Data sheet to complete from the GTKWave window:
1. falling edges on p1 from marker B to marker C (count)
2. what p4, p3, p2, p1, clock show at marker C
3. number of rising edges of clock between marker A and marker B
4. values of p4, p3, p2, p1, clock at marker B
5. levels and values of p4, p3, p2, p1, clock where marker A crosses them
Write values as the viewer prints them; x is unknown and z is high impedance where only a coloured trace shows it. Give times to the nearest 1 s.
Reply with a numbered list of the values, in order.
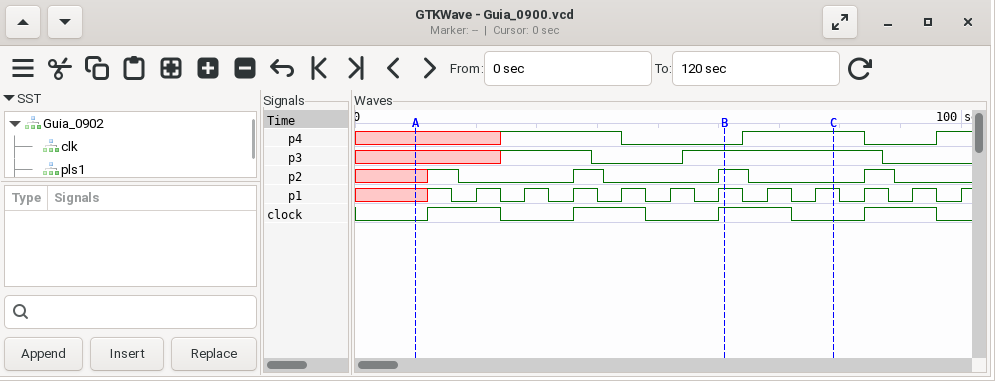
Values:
1. 2
2. p4=1, p3=1, p2=0, p1=1, clock=0
3. 3
4. p4=0, p3=1, p2=1, p1=1, clock=1
5. p4=x, p3=x, p2=x, p1=x, clock=0
